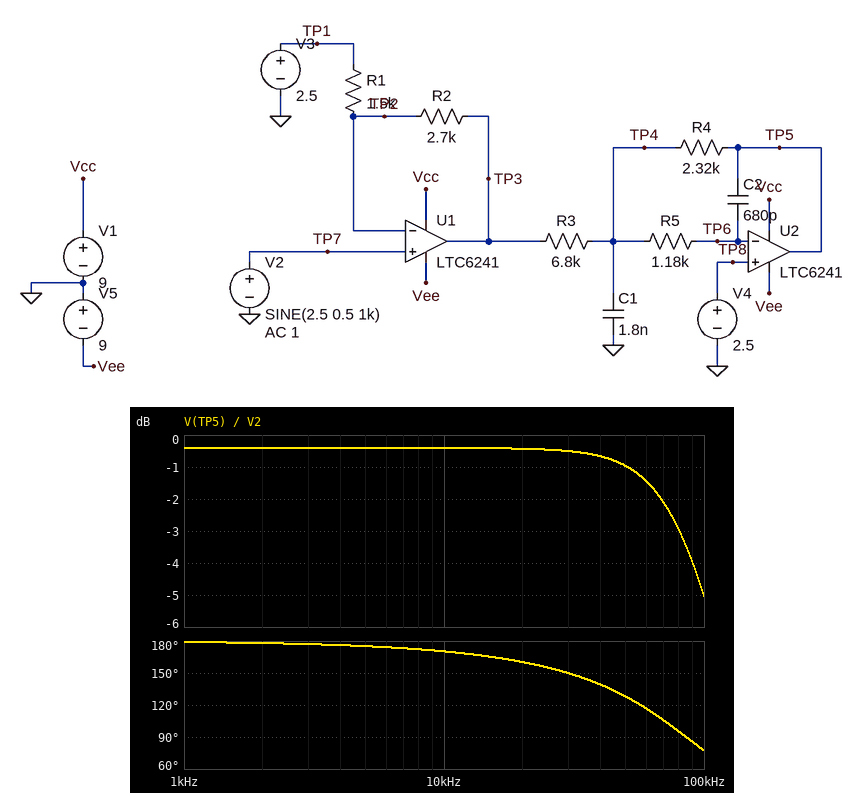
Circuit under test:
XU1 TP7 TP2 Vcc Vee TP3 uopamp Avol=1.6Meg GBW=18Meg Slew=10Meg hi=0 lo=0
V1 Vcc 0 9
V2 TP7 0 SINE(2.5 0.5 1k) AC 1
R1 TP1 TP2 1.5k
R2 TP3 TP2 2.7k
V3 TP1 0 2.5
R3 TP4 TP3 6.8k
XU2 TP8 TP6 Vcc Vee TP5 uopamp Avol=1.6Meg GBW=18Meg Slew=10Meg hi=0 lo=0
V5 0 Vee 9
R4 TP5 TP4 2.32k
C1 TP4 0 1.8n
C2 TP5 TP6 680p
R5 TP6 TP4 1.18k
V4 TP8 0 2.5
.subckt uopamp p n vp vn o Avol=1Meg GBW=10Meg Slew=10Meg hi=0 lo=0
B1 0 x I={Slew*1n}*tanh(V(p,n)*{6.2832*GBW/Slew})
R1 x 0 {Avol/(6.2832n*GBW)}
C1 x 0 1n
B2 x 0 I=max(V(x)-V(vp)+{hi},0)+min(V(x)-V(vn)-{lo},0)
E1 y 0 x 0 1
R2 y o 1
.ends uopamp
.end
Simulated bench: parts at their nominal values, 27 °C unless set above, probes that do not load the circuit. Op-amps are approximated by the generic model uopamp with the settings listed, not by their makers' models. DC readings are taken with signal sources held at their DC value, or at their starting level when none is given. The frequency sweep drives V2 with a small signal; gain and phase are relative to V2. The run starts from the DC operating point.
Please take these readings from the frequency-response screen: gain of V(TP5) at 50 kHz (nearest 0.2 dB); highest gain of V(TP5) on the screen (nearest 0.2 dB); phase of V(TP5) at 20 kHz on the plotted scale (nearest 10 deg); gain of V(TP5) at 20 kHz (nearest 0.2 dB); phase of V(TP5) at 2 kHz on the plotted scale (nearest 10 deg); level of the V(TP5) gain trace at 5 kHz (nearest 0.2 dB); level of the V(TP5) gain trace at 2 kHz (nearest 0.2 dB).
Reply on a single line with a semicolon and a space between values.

-1.0 dB; -0.4 dB; 160 deg; -0.4 dB; 180 deg; -0.4 dB; -0.4 dB
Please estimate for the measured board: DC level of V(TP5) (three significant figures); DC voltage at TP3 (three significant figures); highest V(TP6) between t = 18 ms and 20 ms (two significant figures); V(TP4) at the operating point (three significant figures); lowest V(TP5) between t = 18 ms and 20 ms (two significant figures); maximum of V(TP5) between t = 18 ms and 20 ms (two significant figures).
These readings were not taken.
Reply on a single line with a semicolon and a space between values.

2.50 V; 2.50 V; 2.5 V; 2.50 V; 2.0 V; 3.0 V
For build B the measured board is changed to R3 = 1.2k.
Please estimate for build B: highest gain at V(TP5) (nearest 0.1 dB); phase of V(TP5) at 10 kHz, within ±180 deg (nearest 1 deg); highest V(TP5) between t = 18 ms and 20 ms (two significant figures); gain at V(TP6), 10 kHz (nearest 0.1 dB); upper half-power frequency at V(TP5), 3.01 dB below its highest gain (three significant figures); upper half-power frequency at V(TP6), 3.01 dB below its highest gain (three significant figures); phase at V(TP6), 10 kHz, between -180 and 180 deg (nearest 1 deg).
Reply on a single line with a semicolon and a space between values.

14.7 dB; 166 deg; 5.2 V; -50.6 dB; 50.4 kHz; 219 kHz; 76 deg
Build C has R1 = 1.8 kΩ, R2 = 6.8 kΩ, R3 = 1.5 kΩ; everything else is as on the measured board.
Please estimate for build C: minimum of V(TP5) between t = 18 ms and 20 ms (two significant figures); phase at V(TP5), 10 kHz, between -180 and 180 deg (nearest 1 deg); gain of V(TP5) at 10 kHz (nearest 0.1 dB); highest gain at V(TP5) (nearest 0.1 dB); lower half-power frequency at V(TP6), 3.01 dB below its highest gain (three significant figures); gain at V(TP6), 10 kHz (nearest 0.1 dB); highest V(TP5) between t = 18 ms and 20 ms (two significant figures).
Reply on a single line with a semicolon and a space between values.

-1.2 V; 167 deg; 17.3 dB; 17.4 dB; 36.1 kHz; -47.8 dB; 6.2 V
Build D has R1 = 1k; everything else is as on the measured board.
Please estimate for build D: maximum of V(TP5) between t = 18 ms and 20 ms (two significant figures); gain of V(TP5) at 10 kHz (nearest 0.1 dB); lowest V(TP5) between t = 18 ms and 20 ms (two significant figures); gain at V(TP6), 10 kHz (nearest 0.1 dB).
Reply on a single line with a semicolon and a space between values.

3.1 V; 2.0 dB; 1.9 V; -63.1 dB
